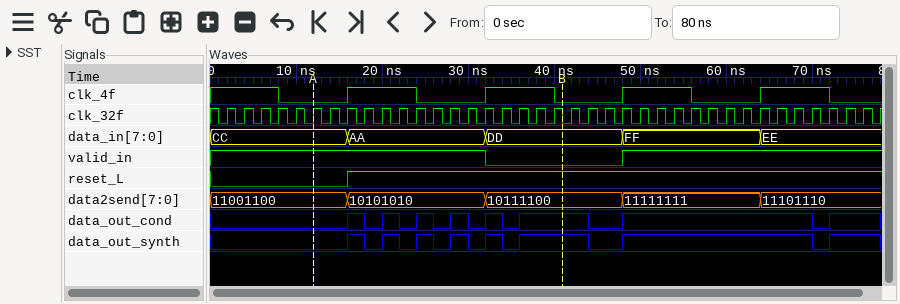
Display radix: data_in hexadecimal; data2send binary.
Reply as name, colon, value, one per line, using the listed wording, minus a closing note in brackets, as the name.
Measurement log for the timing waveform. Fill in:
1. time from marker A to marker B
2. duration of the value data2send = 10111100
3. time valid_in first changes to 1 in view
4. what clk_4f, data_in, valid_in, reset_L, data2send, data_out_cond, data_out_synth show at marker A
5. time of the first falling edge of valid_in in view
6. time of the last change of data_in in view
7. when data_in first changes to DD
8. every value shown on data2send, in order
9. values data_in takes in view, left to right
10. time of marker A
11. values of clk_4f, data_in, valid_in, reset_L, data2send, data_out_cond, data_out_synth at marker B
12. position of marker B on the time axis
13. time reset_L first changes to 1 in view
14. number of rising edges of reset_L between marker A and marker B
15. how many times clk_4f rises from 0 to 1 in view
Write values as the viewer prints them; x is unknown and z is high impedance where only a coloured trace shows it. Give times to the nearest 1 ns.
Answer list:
time from marker A to marker B: 29 ns
duration of the value data2send = 10111100: 16 ns
time valid_in first changes to 1 in view: 48 ns
what clk_4f, data_in, valid_in, reset_L, data2send, data_out_cond, data_out_synth show at marker A: clk_4f=0, data_in=CC, valid_in=1, reset_L=0, data2send=11001100, data_out_cond=0, data_out_synth=0
time of the first falling edge of valid_in in view: 32 ns
time of the last change of data_in in view: 64 ns
when data_in first changes to DD: 32 ns
every value shown on data2send, in order: 11001100, 10101010, 10111100, 11111111, 11101110
values data_in takes in view, left to right: CC, AA, DD, FF, EE
time of marker A: 12 ns
values of clk_4f, data_in, valid_in, reset_L, data2send, data_out_cond, data_out_synth at marker B: clk_4f=0, data_in=DD, valid_in=0, reset_L=1, data2send=10111100, data_out_cond=1, data_out_synth=1
position of marker B on the time axis: 41 ns
time reset_L first changes to 1 in view: 16 ns
number of rising edges of reset_L between marker A and marker B: 1
how many times clk_4f rises from 0 to 1 in view: 4
